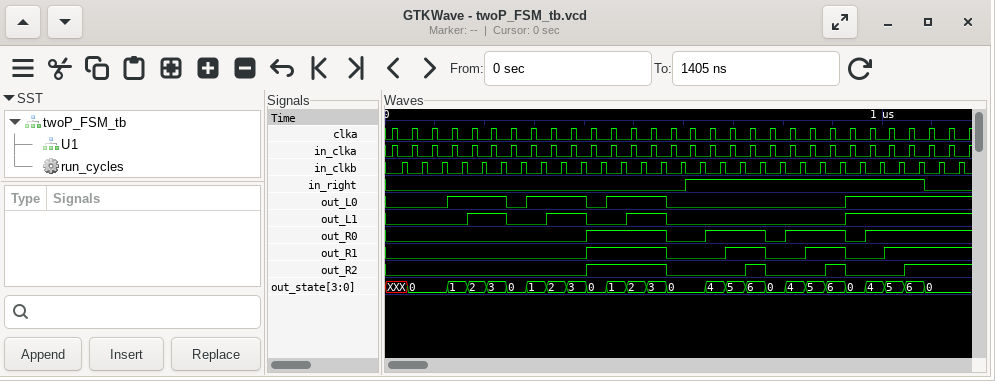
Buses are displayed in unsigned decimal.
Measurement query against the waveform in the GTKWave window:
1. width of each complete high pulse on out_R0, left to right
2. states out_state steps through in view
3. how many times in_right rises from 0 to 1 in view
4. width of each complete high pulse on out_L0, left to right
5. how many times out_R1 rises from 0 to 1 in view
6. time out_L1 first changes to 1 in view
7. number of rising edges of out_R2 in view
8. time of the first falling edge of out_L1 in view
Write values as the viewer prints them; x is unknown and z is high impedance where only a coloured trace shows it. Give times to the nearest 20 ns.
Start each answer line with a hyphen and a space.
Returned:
- 160 ns, 120 ns, 120 ns
- XXX, 0, 1, 2, 3, 0, 1, 2, 3, 0, 1, 2, 3, 0, 4, 5, 6, 0, 4, 5, 6, 0, 4, 5, 6, 0
- 1
- 120 ns, 120 ns, 120 ns
- 4
- 160 ns
- 4
- 240 ns
